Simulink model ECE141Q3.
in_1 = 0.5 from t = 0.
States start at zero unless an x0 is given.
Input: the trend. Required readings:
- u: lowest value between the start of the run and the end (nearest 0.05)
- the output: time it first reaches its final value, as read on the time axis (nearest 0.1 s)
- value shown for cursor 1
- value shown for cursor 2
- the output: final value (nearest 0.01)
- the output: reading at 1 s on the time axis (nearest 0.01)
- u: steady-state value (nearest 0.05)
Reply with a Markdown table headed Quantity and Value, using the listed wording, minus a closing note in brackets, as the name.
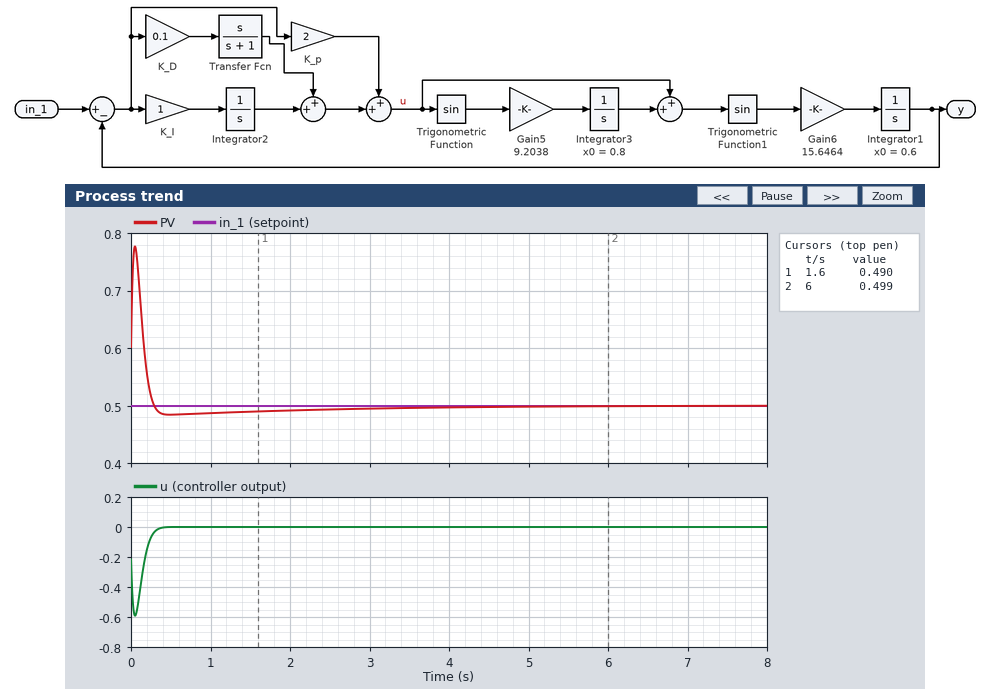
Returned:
| Quantity | Value |
|---|---|
| u: lowest value between the start of the run and the end | -0.60 |
| the output: time it first reaches its final value, as read on the time axis | 0.3 s |
| value shown for cursor 1 | 0.490 |
| value shown for cursor 2 | 0.499 |
| the output: final value | 0.50 |
| the output: reading at 1 s on the time axis | 0.49 |
| u: steady-state value | 0.00 |
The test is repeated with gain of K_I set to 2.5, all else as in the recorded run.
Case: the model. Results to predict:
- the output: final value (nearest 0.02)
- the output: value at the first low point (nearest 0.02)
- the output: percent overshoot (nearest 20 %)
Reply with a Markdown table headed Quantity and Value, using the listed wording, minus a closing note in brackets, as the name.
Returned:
| Quantity | Value |
|---|---|
| the output: final value | 0.50 |
| the output: value at the first low point | 0.46 |
| the output: percent overshoot | 40 % |
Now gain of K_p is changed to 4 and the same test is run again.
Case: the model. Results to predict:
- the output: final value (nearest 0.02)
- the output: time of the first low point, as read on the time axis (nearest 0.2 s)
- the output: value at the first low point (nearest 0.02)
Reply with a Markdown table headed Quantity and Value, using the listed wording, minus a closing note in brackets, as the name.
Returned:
| Quantity | Value |
|---|---|
| the output: final value | 0.50 |
| the output: time of the first low point, as read on the time axis | 0.8 s |
| the output: value at the first low point | 0.50 |
